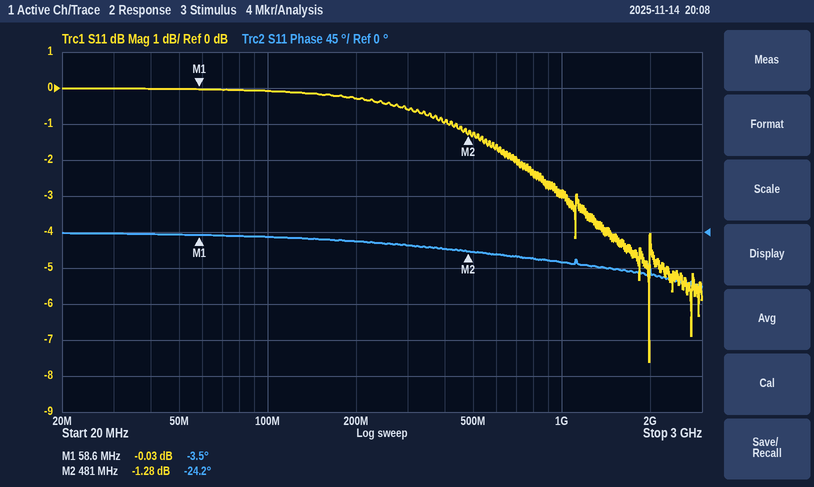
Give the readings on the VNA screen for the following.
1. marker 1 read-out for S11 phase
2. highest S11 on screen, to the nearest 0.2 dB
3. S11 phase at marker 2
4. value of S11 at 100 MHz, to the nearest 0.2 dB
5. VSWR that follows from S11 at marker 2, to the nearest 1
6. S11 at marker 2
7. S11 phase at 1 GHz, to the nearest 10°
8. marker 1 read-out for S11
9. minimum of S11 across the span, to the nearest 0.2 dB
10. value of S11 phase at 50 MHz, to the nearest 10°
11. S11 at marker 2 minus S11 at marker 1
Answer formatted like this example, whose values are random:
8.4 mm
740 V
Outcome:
-3.5°
0.0 dB
-24.2°
0.0 dB
14
-1.28 dB
-40°
-0.03 dB
-7.6 dB
0°
-1.25 dB
